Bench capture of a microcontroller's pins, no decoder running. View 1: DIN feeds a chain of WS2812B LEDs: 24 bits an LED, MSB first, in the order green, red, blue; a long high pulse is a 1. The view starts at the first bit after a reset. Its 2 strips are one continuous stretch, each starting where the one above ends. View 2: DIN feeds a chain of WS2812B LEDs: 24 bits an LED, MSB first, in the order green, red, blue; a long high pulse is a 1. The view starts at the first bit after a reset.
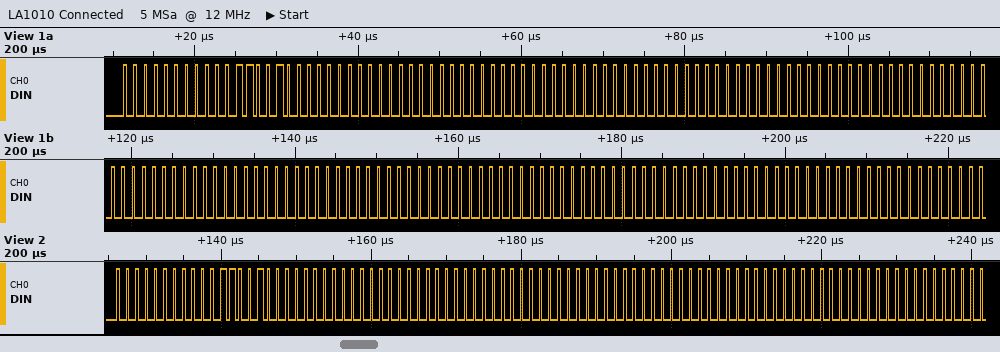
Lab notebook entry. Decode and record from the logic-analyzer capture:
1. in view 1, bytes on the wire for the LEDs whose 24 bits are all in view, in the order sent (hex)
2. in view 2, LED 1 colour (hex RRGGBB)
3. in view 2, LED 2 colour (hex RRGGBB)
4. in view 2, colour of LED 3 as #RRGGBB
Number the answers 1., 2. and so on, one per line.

1. 00 19 00 00 00 00 00 00 00 00 00 00 00 00 00 00 00 00 00 00 00
2. #190000
3. #000000
4. #000000
